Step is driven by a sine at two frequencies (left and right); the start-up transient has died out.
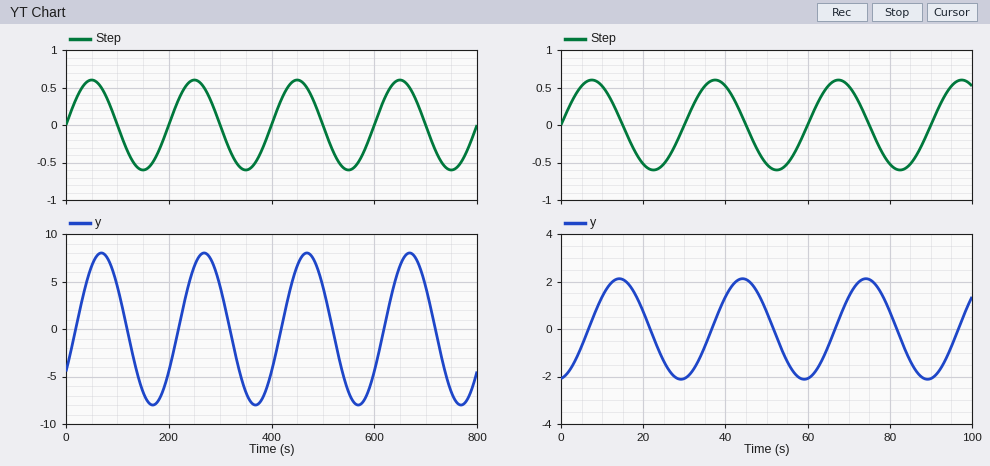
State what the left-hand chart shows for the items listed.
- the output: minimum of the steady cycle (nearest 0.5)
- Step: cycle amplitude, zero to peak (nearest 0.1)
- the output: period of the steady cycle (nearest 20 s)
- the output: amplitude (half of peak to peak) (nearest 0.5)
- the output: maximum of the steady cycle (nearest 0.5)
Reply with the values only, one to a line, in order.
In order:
-8.0
0.6
200 s
8.0
8.0
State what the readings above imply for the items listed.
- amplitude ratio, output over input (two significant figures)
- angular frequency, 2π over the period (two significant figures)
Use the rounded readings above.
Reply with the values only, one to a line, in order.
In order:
13
0.031 rad/s
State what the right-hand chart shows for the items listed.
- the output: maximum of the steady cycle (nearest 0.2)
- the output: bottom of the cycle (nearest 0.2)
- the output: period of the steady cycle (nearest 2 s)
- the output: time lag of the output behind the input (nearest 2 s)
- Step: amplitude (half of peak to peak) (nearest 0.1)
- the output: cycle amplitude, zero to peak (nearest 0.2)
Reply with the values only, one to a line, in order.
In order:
2.2
-2.2
30 s
6 s
0.6
2.2
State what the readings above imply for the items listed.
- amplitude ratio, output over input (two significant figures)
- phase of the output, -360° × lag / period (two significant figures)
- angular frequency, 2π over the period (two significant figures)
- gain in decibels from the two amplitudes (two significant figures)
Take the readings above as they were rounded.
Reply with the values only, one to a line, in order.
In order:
3.7
-72°
0.21 rad/s
11 dB
